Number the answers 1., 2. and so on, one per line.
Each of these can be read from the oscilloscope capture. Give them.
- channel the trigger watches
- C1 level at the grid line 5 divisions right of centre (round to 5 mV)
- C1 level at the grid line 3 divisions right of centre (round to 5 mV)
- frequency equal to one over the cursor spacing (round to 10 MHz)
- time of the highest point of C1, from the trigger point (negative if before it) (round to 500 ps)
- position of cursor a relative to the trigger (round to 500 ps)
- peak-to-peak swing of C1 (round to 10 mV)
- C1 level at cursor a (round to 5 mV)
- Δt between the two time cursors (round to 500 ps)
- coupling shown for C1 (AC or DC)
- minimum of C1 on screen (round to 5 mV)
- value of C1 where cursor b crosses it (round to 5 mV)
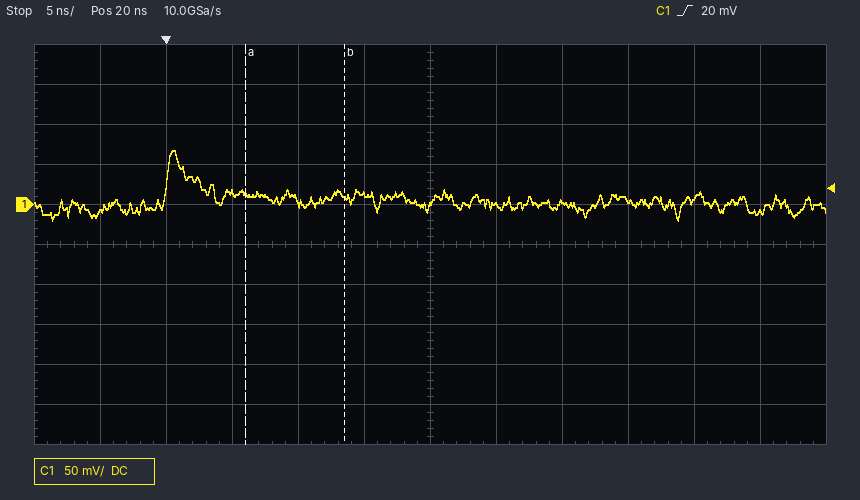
1. C1
2. -10 mV
3. 5 mV
4. 130 MHz
5. +500 ps
6. +6.0 ns
7. 90 mV
8. 15 mV
9. 7.5 ns
10. DC
11. -20 mV
12. 10 mV
